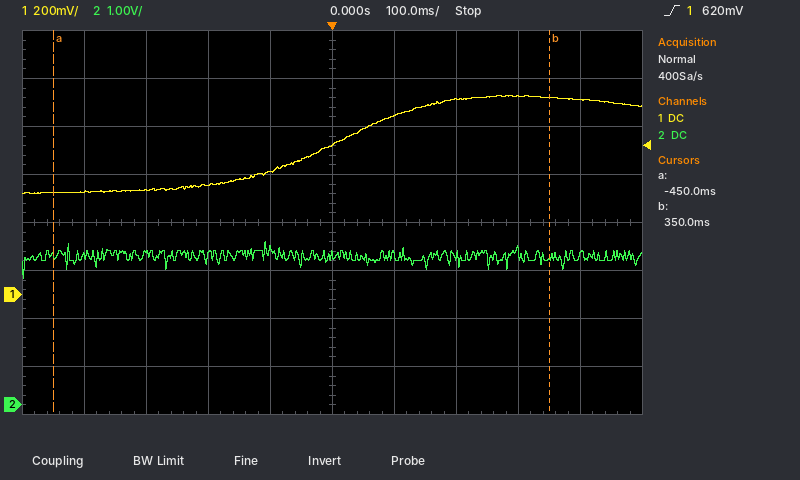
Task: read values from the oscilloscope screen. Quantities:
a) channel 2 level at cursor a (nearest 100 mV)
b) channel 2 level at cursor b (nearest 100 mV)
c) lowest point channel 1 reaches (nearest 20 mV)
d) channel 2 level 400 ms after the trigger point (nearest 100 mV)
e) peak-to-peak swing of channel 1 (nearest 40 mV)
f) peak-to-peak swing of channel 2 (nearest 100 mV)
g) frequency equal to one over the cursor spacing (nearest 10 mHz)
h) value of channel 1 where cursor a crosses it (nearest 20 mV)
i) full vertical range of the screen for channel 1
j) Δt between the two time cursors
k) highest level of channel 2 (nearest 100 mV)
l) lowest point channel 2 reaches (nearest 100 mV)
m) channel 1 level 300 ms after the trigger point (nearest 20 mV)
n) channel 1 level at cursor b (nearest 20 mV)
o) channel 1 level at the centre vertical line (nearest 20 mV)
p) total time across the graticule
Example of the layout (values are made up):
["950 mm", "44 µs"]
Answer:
["3.1 V", "3.1 V", "420 mV", "3.1 V", "400 mV", "800 mV", "1.25 Hz", "420 mV", "1.6 V", "800 ms", "3.4 V", "2.6 V", "820 mV", "820 mV", "620 mV", "1 s"]
